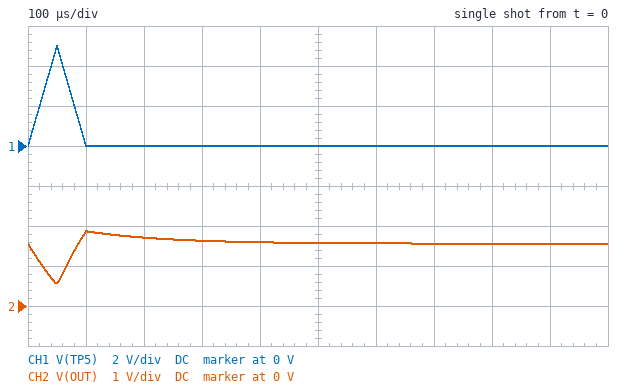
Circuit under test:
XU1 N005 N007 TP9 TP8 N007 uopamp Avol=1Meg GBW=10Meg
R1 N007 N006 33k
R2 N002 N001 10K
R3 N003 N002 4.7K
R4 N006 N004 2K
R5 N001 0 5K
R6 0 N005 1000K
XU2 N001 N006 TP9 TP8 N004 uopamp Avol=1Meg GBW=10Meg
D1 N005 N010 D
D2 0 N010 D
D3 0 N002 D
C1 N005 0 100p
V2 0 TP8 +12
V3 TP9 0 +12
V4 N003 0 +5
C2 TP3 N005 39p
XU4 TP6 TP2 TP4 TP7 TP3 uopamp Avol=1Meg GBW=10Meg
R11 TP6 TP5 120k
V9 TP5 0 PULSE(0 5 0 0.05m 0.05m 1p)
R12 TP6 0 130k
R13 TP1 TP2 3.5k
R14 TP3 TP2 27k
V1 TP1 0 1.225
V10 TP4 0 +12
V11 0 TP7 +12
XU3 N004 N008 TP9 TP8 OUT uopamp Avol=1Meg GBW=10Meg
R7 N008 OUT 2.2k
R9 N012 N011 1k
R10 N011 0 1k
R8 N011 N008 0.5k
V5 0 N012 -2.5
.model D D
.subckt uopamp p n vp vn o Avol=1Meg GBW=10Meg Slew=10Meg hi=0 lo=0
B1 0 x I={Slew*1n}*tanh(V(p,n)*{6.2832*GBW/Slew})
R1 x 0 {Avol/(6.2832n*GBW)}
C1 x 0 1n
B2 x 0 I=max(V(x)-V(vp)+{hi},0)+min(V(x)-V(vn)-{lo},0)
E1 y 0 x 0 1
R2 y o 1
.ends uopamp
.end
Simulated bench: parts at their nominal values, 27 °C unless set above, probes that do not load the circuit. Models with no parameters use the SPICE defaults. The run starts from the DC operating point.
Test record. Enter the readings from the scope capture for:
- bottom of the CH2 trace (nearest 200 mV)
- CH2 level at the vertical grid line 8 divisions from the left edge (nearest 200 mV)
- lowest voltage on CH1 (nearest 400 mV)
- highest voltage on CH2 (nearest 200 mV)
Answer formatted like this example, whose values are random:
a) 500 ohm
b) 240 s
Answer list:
a) 600 mV
b) 1.6 V
c) 0 V
d) 1.8 V
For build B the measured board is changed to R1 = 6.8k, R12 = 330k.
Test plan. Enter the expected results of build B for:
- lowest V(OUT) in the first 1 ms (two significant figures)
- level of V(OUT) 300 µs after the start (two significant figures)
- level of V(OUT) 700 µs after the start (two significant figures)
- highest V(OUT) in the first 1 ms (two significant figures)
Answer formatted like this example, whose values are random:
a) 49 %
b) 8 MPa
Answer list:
a) -2.5 V
b) 3.0 V
c) 2.5 V
d) 4.4 V
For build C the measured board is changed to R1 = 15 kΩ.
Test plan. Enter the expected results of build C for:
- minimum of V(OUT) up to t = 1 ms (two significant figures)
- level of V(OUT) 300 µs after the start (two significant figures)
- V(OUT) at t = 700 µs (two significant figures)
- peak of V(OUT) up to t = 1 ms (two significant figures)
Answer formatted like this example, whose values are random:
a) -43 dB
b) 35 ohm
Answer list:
a) -320 mV
b) 2.0 V
c) 1.9 V
d) 2.5 V
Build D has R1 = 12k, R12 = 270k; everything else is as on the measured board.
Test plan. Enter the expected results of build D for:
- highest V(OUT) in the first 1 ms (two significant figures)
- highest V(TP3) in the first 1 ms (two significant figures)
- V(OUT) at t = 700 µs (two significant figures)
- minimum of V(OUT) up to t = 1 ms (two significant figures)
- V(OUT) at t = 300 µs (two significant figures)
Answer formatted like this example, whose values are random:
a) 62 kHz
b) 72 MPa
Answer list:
a) 3.0 V
b) 12 V
c) 2.0 V
d) -840 mV
e) 2.2 V
